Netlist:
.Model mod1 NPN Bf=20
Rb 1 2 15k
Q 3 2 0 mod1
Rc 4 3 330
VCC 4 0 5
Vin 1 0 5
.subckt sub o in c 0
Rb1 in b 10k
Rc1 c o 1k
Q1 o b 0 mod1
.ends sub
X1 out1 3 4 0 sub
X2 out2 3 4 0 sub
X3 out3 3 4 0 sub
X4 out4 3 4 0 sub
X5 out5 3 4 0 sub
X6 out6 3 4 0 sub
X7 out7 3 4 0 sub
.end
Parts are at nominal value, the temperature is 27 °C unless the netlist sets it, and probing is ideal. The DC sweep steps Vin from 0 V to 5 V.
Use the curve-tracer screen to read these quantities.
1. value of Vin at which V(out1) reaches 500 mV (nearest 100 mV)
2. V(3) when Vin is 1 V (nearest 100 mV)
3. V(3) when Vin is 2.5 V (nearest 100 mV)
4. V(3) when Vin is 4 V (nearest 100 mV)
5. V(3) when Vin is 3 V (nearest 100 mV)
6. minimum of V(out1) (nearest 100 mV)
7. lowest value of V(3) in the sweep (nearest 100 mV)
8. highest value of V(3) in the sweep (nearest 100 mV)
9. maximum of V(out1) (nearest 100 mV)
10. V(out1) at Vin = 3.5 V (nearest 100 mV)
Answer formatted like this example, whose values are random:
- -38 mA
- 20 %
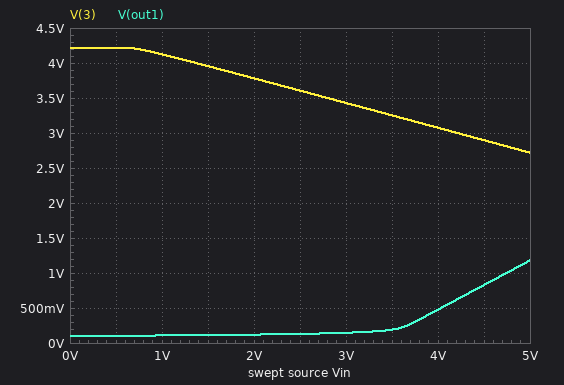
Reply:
- 4.0 V
- 4.1 V
- 3.6 V
- 3.1 V
- 3.4 V
- 100 mV
- 2.7 V
- 4.2 V
- 1.2 V
- 200 mV
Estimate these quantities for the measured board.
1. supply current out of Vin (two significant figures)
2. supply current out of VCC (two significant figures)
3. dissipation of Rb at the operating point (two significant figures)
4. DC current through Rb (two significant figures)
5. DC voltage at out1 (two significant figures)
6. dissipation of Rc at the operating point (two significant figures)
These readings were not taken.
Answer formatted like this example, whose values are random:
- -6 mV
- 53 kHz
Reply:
- 280 µA
- 34 mA
- 1.2 mW
- 280 µA
- 1.2 V
- 16 mW
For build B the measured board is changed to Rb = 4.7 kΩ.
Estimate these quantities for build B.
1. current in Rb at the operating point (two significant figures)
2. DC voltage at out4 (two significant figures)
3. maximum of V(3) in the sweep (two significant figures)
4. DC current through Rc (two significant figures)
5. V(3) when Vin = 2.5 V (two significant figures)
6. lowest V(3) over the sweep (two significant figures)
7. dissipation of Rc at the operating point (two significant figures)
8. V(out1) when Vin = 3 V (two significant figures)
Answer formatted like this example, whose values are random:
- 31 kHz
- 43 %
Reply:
- 880 µA
- 5.0 V
- 4.2 V
- 15 mA
- 2.3 V
- 120 mV
- 72 mW
- 3.1 V
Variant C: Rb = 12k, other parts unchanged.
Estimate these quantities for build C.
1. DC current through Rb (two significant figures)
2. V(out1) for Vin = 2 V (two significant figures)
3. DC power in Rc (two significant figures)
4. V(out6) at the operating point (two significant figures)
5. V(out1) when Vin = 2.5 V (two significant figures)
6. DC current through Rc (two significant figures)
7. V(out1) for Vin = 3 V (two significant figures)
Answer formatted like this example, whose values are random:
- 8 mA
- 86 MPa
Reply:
- 350 µA
- 130 mV
- 21 mW
- 1.9 V
- 140 mV
- 8.0 mA
- 200 mV
